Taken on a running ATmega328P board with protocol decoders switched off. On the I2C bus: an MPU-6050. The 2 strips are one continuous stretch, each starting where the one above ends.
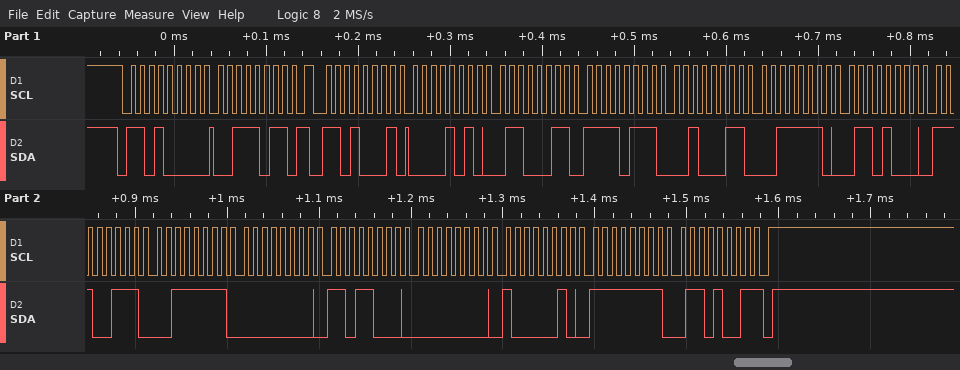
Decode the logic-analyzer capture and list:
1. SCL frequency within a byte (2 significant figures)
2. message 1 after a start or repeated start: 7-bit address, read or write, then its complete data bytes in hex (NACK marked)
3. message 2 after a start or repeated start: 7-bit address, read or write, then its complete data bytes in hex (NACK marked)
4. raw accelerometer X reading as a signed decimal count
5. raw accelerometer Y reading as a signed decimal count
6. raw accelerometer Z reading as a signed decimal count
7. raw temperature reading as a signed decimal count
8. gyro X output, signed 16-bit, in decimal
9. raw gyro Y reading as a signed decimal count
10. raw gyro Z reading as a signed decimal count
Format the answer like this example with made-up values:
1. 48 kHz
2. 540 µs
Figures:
1. 100 kHz
2. 0x68 write: 3B
3. 0x68 read: 0A 63 F7 23 3E 68 E7 3F 00 D8 00 82 FF 69 NACK
4. 2659
5. -2269
6. 15976
7. -6337
8. 216
9. 130
10. -151
